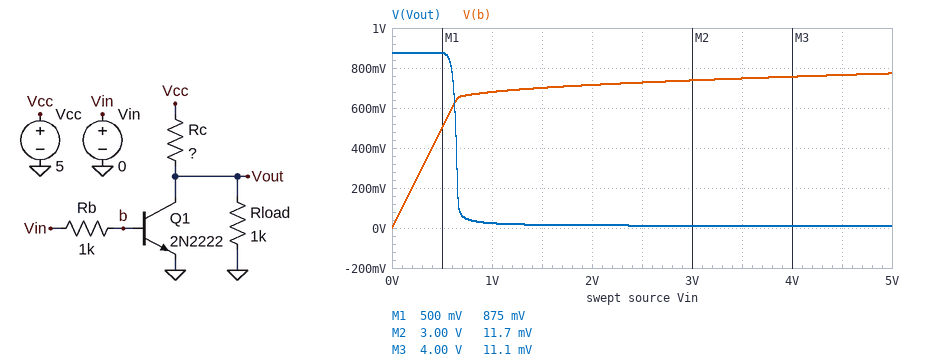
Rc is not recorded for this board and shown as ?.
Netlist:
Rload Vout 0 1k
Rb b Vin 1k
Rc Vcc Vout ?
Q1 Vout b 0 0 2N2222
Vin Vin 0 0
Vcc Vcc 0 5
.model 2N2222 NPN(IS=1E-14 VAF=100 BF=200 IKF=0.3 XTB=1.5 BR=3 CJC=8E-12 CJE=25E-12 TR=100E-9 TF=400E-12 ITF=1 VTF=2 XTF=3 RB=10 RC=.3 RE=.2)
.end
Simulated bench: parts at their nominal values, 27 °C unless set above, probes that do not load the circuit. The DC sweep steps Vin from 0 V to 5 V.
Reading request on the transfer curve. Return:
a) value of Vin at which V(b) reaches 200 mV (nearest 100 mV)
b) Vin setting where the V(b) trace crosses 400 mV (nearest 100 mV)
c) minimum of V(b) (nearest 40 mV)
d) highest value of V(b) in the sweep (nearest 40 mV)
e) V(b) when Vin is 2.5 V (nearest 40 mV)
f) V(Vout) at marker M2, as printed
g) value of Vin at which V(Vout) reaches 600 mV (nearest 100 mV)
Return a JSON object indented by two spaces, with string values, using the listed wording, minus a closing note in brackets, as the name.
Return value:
{
  "value of Vin at which V(b) reaches 200 mV": "200 mV",
  "Vin setting where the V(b) trace crosses 400 mV": "400 mV",
  "minimum of V(b)": "0 V",
  "highest value of V(b) in the sweep": "760 mV",
  "V(b) when Vin is 2.5 V": "720 mV",
  "V(Vout) at marker M2, as printed": "11.7 mV",
  "value of Vin at which V(Vout) reaches 600 mV": "600 mV"
}
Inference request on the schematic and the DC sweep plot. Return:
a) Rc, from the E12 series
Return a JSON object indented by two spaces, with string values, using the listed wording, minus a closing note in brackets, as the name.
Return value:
{
  "Rc, from the E12 series": "4.7 kΩ"
}
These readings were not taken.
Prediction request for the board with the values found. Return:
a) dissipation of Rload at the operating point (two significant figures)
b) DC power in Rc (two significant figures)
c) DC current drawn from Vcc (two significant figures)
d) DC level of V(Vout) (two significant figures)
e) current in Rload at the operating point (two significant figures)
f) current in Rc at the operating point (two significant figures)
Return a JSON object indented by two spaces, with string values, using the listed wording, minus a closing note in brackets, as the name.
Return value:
{
  "dissipation of Rload at the operating point": "770 µW",
  "DC power in Rc": "3.6 mW",
  "DC current drawn from Vcc": "880 µA",
  "DC level of V(Vout)": "880 mV",
  "current in Rload at the operating point": "880 µA",
  "current in Rc at the operating point": "880 µA"
}
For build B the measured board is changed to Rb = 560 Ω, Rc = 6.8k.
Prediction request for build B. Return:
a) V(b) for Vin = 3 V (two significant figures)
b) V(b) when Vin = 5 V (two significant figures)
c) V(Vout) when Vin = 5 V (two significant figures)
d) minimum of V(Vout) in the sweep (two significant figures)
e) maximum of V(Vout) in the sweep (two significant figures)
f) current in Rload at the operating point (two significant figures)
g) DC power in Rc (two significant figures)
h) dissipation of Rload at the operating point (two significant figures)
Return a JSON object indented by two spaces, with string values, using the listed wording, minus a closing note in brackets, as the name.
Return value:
{
  "V(b) for Vin = 3 V": "770 mV",
  "V(b) when Vin = 5 V": "820 mV",
  "V(Vout) when Vin = 5 V": "11 mV",
  "minimum of V(Vout) in the sweep": "10 mV",
  "maximum of V(Vout) in the sweep": "640 mV",
  "current in Rload at the operating point": "640 µA",
  "DC power in Rc": "2.8 mW",
  "dissipation of Rload at the operating point": "410 µW"
}
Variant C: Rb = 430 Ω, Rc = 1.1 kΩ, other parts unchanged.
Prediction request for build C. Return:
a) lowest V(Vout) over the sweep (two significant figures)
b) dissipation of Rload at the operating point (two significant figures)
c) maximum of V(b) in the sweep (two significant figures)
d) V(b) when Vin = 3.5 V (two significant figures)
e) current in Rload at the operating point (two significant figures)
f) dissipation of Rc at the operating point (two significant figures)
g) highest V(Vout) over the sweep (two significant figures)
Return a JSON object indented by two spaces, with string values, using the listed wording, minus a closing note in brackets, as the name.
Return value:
{
  "lowest V(Vout) over the sweep": "16 mV",
  "dissipation of Rload at the operating point": "5.7 mW",
  "maximum of V(b) in the sweep": "850 mV",
  "V(b) when Vin = 3.5 V": "810 mV",
  "current in Rload at the operating point": "2.4 mA",
  "dissipation of Rc at the operating point": "6.2 mW",
  "highest V(Vout) over the sweep": "2.4 V"
}
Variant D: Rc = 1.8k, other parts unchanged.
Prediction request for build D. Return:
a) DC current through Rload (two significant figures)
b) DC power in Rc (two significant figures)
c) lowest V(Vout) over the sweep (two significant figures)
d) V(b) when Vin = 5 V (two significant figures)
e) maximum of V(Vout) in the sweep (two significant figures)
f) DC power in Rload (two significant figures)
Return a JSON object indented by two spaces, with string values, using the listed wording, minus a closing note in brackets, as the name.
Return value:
{
  "DC current through Rload": "1.8 mA",
  "DC power in Rc": "5.7 mW",
  "lowest V(Vout) over the sweep": "14 mV",
  "V(b) when Vin = 5 V": "780 mV",
  "maximum of V(Vout) in the sweep": "1.8 V",
  "DC power in Rload": "3.2 mW"
}
